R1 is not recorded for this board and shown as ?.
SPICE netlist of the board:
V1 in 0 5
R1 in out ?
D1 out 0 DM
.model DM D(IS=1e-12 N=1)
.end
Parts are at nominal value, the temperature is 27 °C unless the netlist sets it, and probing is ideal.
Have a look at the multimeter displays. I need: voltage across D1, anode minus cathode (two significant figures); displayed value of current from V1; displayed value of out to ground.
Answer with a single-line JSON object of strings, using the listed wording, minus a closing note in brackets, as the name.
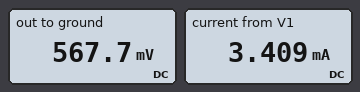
{"voltage across D1, anode minus cathode": "570 mV", "displayed value of current from V1": "3.409 mA", "displayed value of out to ground": "567.7 mV"}
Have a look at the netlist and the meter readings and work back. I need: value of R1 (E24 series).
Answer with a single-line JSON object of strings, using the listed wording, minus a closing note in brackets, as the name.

{"value of R1": "1.3 kΩ"}
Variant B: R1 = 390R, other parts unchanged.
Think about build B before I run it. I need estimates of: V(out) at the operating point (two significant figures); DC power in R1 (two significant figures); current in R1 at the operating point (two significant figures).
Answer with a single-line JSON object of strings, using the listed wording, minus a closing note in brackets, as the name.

{"V(out) at the operating point": "600 mV", "DC power in R1": "50 mW", "current in R1 at the operating point": "11 mA"}
